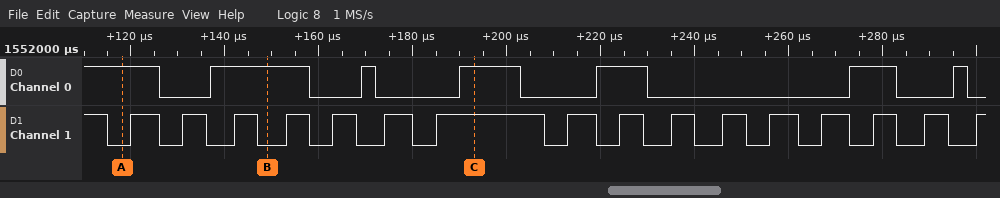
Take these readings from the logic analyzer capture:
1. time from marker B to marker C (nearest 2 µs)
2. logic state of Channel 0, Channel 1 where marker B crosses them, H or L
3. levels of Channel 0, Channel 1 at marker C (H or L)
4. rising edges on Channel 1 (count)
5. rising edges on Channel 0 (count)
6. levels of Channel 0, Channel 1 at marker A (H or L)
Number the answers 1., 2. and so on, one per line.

1. 44 µs
2. Channel 0=H, Channel 1=L
3. Channel 0=H, Channel 1=H
4. 16
5. 6
6. Channel 0=H, Channel 1=L
